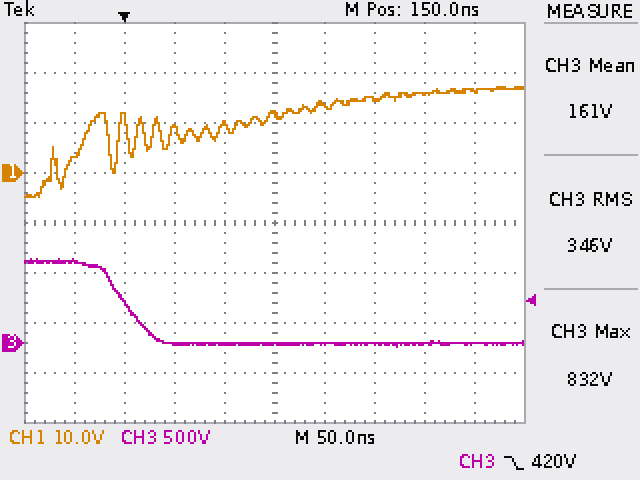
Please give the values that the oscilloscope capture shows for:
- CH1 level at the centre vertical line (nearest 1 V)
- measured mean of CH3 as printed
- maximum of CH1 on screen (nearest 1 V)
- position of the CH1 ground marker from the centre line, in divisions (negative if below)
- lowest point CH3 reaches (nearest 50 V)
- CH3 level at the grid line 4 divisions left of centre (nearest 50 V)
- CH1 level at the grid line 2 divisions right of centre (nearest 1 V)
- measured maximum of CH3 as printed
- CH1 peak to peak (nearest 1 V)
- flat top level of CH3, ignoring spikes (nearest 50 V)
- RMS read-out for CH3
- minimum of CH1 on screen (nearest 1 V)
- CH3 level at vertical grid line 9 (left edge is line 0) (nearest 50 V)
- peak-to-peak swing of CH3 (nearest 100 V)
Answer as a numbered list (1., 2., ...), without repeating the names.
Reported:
1. 12 V
2. 161 V
3. 17 V
4. +1.0 div
5. -50 V
6. 800 V
7. 15 V
8. 832 V
9. 22 V
10. 800 V
11. 346 V
12. -5 V
13. 0 V
14. 900 V
